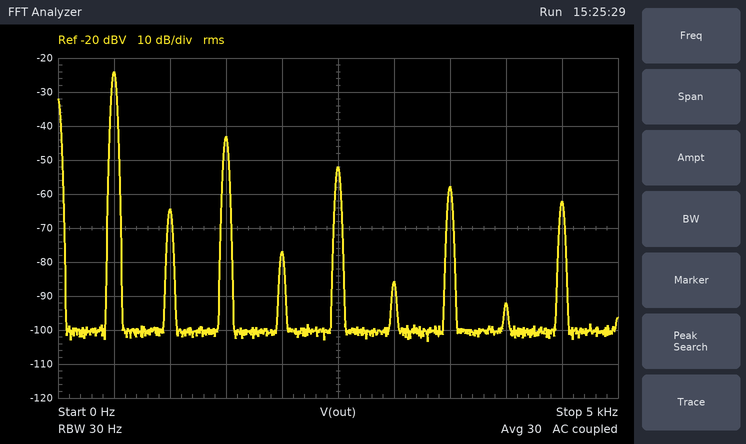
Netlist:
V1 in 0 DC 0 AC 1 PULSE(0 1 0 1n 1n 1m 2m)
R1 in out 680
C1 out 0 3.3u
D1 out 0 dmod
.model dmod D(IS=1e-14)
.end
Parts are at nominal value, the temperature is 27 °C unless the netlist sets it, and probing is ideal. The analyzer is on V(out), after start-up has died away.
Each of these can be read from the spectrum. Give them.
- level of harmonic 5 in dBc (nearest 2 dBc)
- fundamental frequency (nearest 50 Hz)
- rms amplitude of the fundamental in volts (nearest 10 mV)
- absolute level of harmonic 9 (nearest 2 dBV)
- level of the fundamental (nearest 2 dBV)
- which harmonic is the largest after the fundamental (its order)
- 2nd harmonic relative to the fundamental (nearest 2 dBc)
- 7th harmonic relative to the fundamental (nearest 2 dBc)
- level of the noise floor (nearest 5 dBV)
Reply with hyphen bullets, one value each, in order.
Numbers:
- -28 dBc
- 500 Hz
- 60 mV
- -62 dBV
- -24 dBV
- 3
- -40 dBc
- -34 dBc
- -100 dBV
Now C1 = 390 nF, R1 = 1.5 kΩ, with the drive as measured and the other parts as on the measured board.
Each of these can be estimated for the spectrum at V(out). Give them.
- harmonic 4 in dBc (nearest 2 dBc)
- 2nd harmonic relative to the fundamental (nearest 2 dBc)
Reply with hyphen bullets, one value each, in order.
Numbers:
- -44 dBc
- -18 dBc
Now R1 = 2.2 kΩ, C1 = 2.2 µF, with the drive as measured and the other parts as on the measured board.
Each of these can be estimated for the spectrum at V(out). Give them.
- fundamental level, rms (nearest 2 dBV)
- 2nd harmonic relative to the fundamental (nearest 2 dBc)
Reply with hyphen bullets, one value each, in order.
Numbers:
- -30 dBV
- -50 dBc
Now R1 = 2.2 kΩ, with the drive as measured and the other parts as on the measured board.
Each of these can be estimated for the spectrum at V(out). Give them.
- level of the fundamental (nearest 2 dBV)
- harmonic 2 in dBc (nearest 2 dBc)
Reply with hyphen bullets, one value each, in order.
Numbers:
- -34 dBV
- -58 dBc
